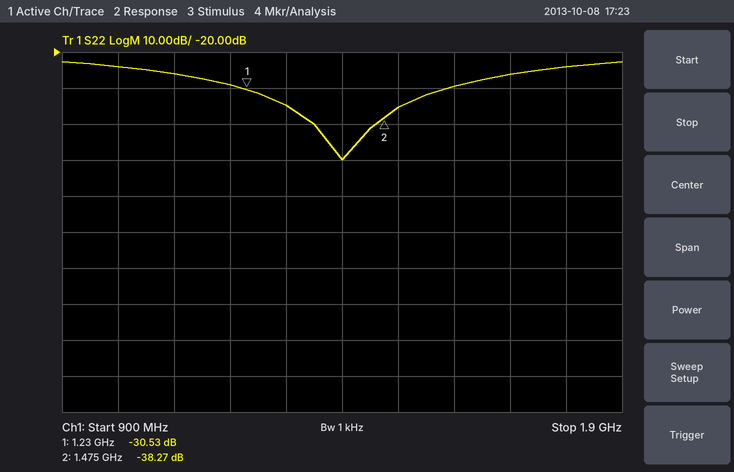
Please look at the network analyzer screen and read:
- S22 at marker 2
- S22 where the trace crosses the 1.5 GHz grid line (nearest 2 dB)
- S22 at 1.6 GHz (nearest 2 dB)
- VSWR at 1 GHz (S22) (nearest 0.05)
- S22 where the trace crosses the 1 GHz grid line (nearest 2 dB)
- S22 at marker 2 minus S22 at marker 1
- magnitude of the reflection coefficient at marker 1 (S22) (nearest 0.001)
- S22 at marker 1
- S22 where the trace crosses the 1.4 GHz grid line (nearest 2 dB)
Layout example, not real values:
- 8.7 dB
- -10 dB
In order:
- -38.27 dB
- -36 dB
- -30 dB
- 1.15
- -24 dB
- -7.74 dB
- 0.030
- -30.53 dB
- -50 dB
